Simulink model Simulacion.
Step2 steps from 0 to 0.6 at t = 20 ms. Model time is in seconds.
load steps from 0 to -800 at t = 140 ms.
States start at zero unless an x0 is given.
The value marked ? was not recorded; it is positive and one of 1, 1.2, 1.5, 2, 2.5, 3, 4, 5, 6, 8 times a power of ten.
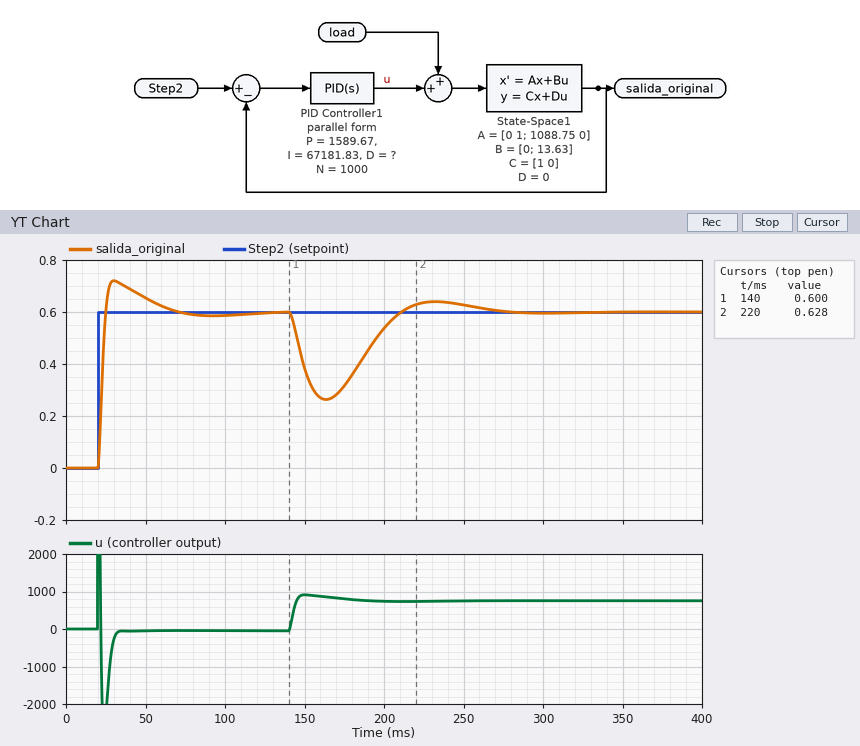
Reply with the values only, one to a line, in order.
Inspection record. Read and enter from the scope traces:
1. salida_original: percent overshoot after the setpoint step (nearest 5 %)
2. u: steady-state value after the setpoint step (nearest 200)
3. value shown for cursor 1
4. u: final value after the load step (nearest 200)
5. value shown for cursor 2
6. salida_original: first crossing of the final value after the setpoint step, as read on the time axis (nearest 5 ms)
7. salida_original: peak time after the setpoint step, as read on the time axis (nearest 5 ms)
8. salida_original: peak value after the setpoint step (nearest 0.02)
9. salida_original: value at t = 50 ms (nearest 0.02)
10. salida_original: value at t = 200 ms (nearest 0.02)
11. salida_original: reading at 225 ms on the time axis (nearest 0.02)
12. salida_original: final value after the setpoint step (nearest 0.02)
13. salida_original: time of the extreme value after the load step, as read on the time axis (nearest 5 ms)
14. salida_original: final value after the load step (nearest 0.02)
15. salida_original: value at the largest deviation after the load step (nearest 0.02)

20 %
0
0.600
800
0.628
25 ms
30 ms
0.72
0.66
0.54
0.64
0.60
165 ms
0.60
0.26
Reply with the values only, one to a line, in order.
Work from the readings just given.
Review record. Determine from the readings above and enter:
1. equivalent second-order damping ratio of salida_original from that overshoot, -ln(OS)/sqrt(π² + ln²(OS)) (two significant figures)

0.46
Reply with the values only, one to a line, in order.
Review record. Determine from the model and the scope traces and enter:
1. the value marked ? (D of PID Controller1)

25
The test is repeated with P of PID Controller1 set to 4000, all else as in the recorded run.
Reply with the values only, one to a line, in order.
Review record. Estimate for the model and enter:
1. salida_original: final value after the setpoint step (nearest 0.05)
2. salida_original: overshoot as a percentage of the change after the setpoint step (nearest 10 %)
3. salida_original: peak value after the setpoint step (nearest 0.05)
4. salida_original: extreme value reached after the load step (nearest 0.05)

0.60
30 %
0.80
0.40
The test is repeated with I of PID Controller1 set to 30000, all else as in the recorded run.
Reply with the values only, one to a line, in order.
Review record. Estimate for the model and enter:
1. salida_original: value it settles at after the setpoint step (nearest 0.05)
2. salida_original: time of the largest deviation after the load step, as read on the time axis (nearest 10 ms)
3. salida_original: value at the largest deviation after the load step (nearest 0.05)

0.60
170 ms
0.20
